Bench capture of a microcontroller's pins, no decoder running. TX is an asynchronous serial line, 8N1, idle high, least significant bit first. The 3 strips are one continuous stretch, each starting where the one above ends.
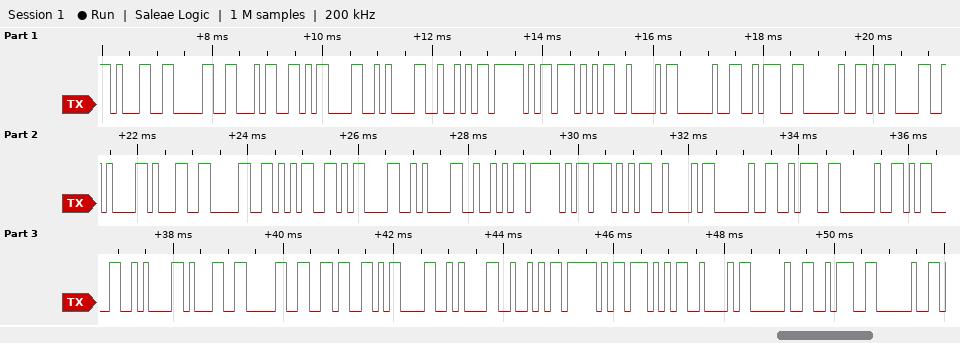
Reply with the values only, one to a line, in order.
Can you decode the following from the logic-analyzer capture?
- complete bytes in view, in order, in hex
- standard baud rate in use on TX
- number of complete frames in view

31 30 34 0D 0A 52 5F 57 42 20 3A 20 0D 0A 31 30 35 0D 0A 52 5F 57 42 20 3A 20 0D 0A 31 30 36 0D 0A 52 5F 57 42 20 3A 20
9600 baud
40
